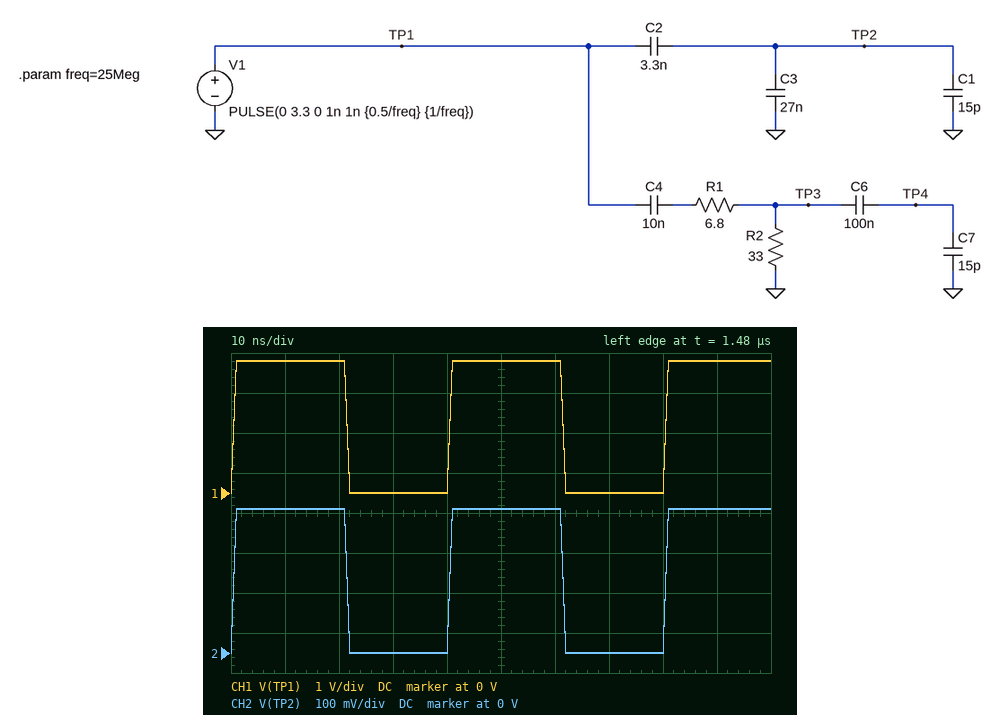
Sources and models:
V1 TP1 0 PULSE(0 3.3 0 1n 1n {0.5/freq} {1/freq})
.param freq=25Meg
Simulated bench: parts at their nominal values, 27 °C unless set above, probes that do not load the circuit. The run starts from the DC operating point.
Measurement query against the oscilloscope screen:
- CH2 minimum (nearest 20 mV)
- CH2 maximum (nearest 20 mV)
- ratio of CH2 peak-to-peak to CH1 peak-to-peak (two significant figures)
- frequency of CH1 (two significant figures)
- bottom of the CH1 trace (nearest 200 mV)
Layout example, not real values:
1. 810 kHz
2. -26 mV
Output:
1. 0 V
2. 360 mV
3. 0.11
4. 25 MHz
5. 0 V
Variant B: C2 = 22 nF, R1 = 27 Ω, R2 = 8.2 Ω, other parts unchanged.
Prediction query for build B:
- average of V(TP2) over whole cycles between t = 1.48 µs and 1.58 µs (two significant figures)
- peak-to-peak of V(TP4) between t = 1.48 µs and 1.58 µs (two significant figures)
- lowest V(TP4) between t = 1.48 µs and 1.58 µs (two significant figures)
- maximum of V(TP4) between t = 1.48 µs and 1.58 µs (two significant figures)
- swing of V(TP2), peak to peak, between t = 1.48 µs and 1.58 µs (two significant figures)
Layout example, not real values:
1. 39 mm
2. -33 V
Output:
1. 780 mV
2. 790 mV
3. -410 mV
4. 380 mV
5. 1.5 V
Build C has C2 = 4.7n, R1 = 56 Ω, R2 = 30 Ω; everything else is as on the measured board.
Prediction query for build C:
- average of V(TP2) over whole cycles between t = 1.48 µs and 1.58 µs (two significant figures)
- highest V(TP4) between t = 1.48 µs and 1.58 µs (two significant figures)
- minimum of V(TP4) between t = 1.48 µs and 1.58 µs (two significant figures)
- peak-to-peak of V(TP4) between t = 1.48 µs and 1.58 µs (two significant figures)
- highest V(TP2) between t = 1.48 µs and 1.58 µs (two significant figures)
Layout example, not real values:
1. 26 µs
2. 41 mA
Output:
1. 260 mV
2. 660 mV
3. -510 mV
4. 1.2 V
5. 490 mV
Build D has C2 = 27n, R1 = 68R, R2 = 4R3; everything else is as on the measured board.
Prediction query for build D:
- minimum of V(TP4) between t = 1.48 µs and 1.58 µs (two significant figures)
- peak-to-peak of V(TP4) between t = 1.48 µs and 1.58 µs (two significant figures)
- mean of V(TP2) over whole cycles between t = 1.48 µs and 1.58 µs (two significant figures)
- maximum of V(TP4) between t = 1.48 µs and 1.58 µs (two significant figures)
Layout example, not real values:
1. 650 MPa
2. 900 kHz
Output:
1. -92 mV
2. 200 mV
3. 870 mV
4. 110 mV
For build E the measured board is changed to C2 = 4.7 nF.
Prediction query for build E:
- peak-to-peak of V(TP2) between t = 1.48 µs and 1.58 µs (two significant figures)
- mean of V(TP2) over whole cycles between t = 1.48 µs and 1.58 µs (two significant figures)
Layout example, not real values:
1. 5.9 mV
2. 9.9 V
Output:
1. 490 mV
2. 260 mV
